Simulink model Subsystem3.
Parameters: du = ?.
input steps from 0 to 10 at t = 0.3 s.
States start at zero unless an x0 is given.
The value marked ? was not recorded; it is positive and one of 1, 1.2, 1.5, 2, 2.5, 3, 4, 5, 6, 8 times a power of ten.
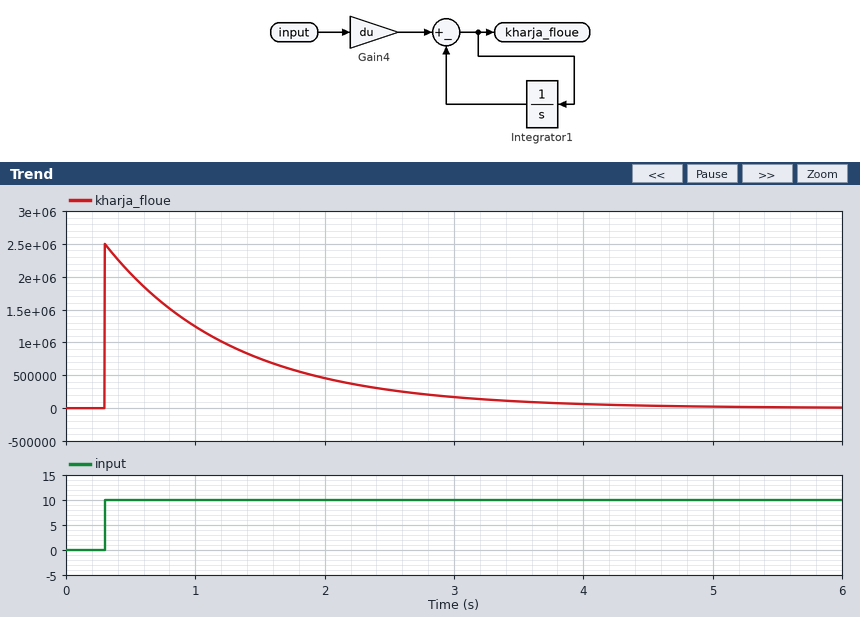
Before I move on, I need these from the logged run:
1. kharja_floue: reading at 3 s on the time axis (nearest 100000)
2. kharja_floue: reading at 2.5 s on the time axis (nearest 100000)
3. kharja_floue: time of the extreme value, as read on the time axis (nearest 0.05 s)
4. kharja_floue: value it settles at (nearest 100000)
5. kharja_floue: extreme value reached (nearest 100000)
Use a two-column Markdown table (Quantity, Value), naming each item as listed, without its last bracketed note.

| Quantity | Value |
|---|---|
| kharja_floue: reading at 3 s on the time axis | 200000 |
| kharja_floue: reading at 2.5 s on the time axis | 300000 |
| kharja_floue: time of the extreme value, as read on the time axis | 0.30 s |
| kharja_floue: value it settles at | 0 |
| kharja_floue: extreme value reached | 2500000 |
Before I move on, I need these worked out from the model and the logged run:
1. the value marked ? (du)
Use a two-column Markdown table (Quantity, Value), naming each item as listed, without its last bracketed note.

| Quantity | Value |
|---|---|
| the value marked ? | 250000 |
